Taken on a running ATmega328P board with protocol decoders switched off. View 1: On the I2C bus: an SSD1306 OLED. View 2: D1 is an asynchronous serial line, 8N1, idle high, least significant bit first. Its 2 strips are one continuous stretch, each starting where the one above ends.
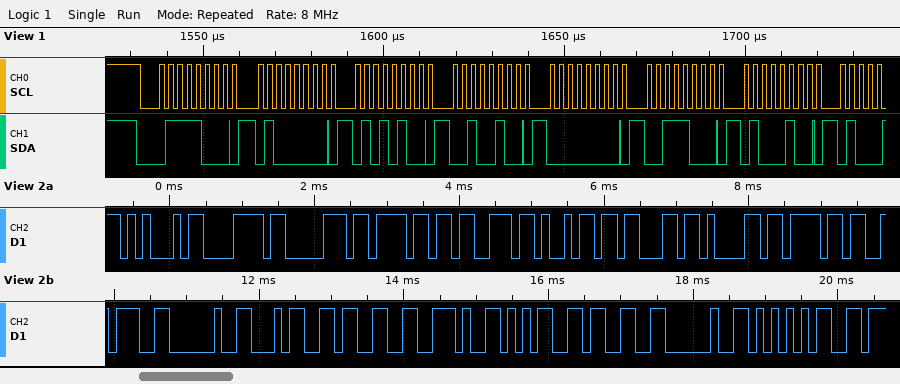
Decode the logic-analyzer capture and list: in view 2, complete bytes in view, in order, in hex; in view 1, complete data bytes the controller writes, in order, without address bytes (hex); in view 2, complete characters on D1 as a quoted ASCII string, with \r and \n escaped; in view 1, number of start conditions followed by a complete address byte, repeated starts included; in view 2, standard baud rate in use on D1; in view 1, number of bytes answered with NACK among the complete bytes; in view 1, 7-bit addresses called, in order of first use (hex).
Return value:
45 78 70 6F 73 69 63 61 6F 3A 20 34 33 2E 35 33 20 55
40 54 24 00 38 44
"Exposicao: 43.53 U"
1
9600 baud
0
0x3C
